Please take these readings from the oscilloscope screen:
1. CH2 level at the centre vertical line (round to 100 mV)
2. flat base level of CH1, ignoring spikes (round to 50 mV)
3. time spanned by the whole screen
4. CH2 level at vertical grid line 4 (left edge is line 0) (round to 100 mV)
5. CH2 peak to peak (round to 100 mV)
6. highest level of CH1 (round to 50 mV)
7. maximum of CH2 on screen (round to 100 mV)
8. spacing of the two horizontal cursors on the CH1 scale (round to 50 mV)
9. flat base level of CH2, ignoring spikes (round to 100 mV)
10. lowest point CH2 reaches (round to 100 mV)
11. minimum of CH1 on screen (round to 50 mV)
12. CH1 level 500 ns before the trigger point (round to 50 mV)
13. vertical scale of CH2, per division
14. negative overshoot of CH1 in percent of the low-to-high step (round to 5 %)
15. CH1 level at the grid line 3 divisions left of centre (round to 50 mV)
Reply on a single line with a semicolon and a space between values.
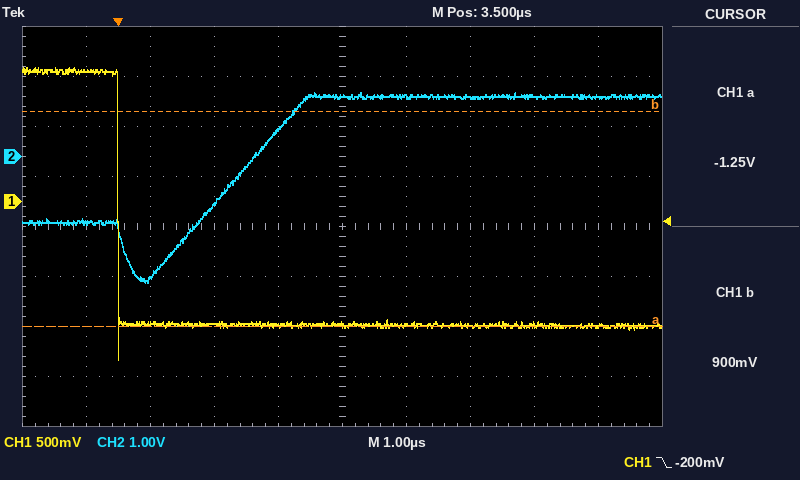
1.2 V; -1.25 V; 10 µs; 500 mV; 3.8 V; 1.35 V; 1.3 V; 2.15 V; -1.3 V; -2.5 V; -1.60 V; 1.30 V; 1 V; 15 %; -1.20 V
